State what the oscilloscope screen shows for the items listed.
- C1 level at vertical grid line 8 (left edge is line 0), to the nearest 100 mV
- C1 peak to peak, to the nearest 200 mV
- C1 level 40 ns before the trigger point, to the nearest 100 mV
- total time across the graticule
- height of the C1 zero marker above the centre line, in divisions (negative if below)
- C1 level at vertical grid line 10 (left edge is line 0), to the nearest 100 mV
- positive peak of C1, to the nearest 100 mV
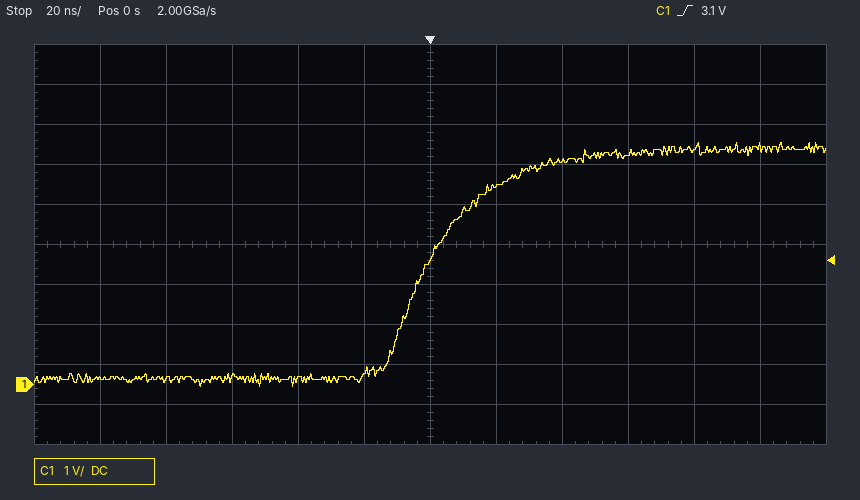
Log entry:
5.6 V
6.0 V
100 mV
240 ns
-3.5 div
5.9 V
6.0 V
